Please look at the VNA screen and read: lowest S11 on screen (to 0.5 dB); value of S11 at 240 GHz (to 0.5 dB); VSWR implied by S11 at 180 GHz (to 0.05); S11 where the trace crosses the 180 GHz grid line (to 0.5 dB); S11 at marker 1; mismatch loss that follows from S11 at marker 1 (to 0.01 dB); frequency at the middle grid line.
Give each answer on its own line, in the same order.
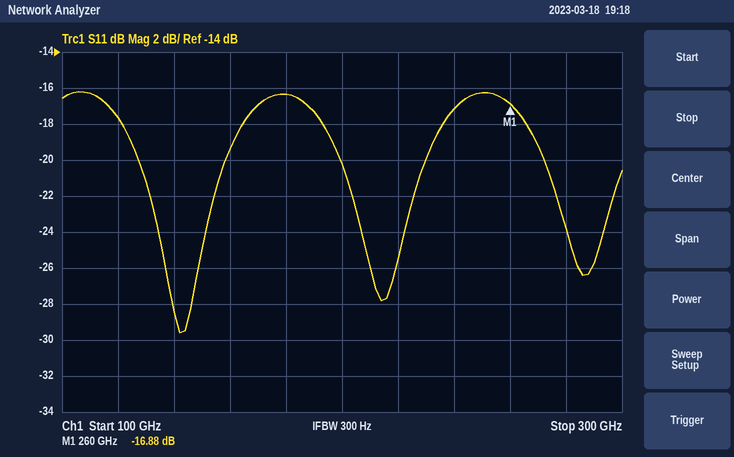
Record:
-29.5 dB
-17.0 dB
1.35
-16.5 dB
-16.88 dB
0.09 dB
200 GHz
